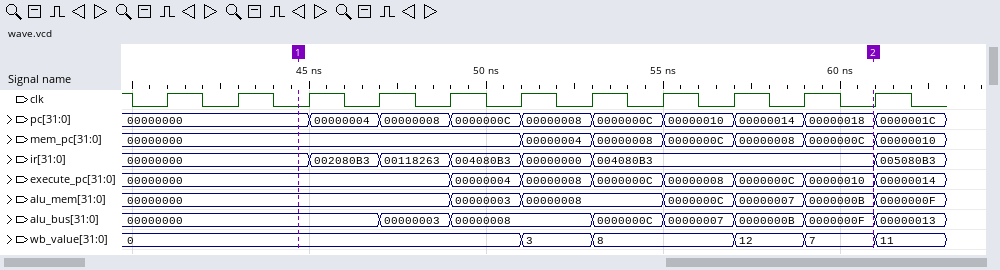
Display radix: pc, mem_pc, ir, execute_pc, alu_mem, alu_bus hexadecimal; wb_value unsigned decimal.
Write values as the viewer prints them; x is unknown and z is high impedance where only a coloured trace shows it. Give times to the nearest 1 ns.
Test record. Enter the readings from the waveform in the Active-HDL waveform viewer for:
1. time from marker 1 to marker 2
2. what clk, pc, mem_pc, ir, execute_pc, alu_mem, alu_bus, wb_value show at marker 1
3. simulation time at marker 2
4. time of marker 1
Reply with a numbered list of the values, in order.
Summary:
1. 16 ns
2. clk=0, pc=00000000, mem_pc=00000000, ir=00000000, execute_pc=00000000, alu_mem=00000000, alu_bus=00000000, wb_value=0
3. 61 ns
4. 45 ns
